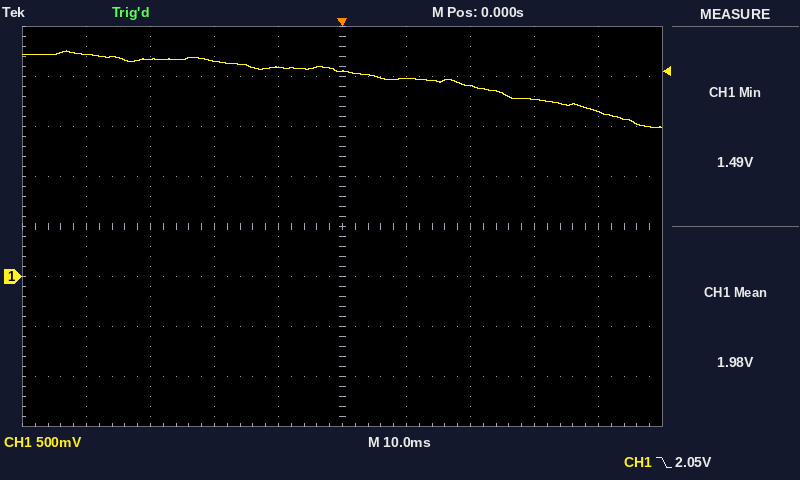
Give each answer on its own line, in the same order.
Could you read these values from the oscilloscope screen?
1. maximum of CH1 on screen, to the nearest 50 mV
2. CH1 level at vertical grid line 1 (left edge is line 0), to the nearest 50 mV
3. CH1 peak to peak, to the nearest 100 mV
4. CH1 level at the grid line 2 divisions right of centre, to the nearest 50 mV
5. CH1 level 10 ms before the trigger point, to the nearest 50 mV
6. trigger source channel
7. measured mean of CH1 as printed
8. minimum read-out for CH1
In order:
2.25 V
2.20 V
800 mV
1.90 V
2.10 V
CH1
1.98 V
1.49 V
